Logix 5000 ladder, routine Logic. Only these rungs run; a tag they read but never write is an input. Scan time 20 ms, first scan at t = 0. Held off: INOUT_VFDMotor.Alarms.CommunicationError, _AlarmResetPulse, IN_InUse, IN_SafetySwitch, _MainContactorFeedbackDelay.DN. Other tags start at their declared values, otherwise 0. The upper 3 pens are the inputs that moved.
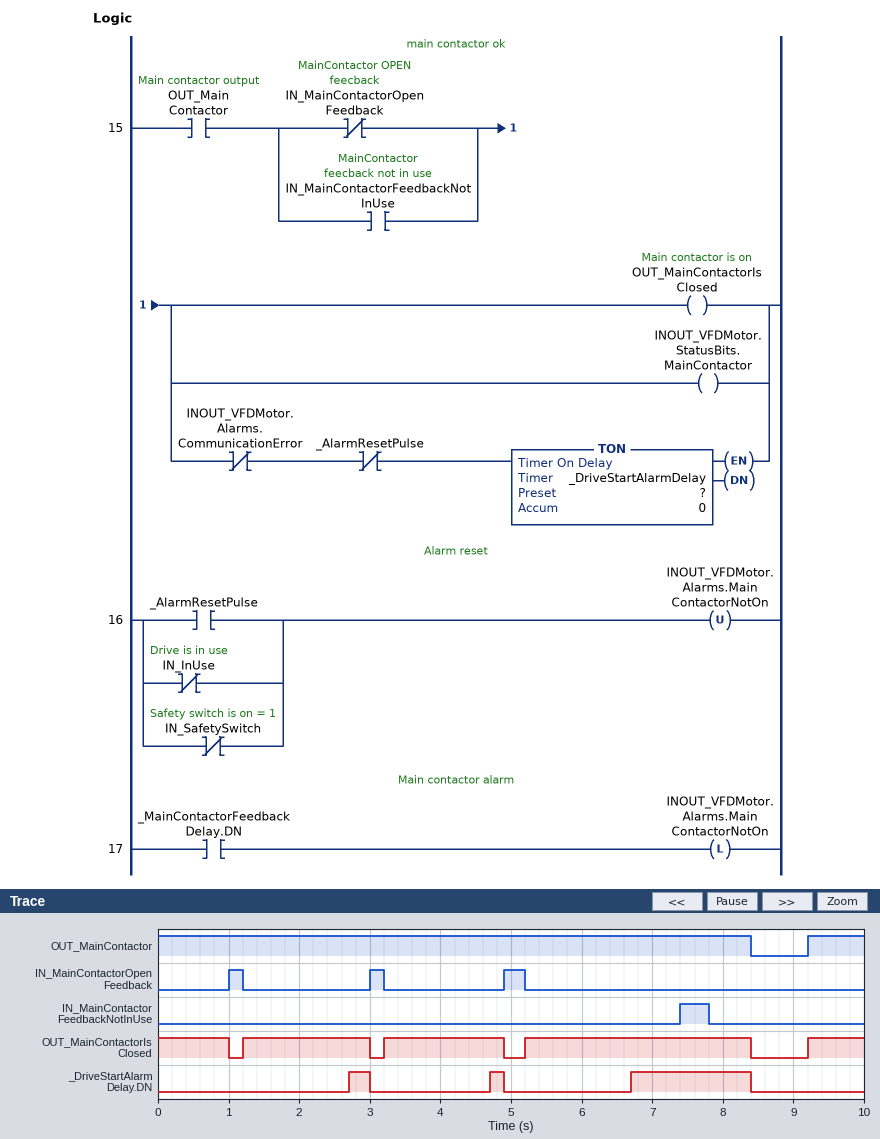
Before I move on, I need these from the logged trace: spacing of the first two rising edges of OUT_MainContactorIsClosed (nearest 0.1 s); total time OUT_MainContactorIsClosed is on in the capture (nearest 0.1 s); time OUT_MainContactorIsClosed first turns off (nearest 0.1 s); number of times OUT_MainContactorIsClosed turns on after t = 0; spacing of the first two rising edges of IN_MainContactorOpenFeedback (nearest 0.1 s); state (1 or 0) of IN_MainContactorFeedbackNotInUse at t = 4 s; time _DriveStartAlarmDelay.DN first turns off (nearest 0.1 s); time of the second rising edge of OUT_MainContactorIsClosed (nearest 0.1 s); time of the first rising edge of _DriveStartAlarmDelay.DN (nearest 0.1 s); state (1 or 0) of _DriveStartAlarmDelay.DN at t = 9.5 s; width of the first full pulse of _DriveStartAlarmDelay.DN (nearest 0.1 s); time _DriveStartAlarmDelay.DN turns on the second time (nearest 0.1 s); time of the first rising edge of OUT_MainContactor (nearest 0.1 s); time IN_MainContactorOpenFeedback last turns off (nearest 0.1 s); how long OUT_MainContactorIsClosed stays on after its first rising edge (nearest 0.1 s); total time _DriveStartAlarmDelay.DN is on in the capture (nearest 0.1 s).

2.0 s
8.5 s
1.0 s
4
2.0 s
0
3.0 s
3.2 s
2.7 s
0
0.3 s
4.7 s
9.2 s
5.2 s
1.8 s
2.2 s
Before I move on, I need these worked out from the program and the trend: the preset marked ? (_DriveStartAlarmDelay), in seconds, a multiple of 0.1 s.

1.5 s
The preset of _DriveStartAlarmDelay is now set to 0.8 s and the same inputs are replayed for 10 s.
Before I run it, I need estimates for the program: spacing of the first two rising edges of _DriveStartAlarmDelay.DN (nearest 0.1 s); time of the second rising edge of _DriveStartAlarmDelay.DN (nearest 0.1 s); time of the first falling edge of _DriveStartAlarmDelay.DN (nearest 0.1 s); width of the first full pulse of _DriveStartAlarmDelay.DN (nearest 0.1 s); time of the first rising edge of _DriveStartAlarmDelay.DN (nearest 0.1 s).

1.2 s
2.0 s
1.0 s
0.2 s
0.8 s
